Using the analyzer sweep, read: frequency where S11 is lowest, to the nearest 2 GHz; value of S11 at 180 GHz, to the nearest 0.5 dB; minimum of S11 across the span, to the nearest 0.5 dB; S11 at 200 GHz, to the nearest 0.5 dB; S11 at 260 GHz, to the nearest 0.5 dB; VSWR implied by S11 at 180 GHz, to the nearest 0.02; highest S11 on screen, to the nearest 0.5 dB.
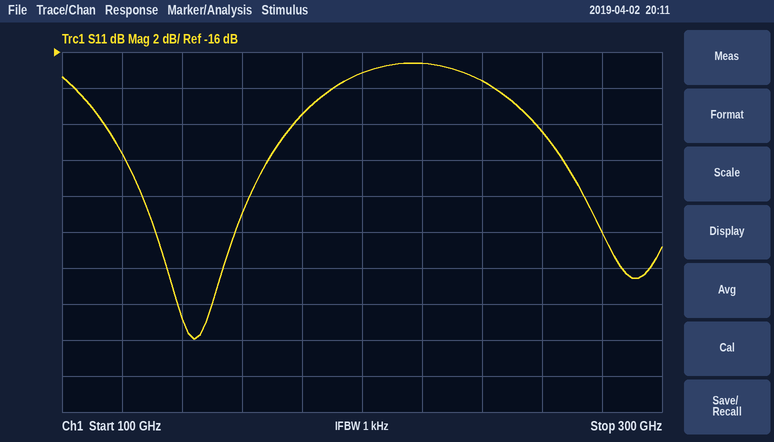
144 GHz
-19.5 dB
-32.0 dB
-17.0 dB
-20.5 dB
1.24
-16.5 dB
